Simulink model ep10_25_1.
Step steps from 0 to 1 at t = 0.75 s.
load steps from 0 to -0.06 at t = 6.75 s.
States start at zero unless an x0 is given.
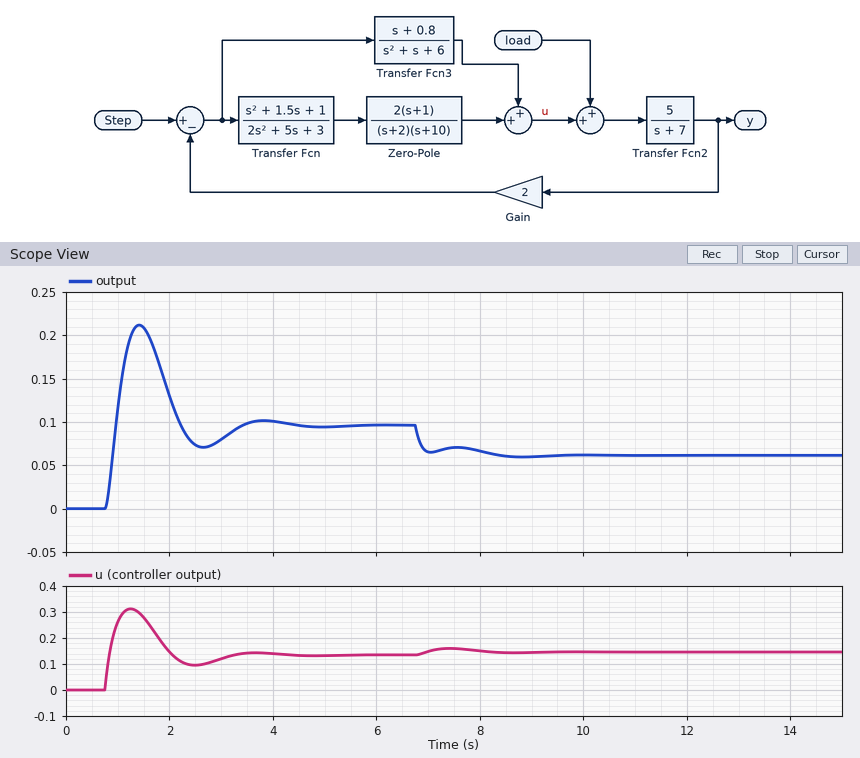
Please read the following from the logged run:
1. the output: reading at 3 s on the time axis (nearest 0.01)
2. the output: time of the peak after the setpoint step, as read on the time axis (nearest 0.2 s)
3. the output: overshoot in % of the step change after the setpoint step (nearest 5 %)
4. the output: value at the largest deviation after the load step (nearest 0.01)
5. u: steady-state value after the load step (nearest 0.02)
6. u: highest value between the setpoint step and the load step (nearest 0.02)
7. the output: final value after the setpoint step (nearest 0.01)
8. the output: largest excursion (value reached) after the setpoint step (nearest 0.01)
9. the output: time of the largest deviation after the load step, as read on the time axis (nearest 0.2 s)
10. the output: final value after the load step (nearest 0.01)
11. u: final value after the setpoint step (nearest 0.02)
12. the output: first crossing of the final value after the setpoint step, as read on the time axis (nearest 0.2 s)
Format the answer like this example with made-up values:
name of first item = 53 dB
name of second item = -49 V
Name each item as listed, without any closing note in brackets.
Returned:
the output: reading at 3 s on the time axis = 0.08
the output: time of the peak after the setpoint step, as read on the time axis = 1.4 s
the output: overshoot in % of the step change after the setpoint step = 120 %
the output: value at the largest deviation after the load step = 0.06
u: steady-state value after the load step = 0.14
u: highest value between the setpoint step and the load step = 0.32
the output: final value after the setpoint step = 0.10
the output: largest excursion (value reached) after the setpoint step = 0.21
the output: time of the largest deviation after the load step, as read on the time axis = 8.8 s
the output: final value after the load step = 0.06
u: final value after the setpoint step = 0.14
the output: first crossing of the final value after the setpoint step, as read on the time axis = 1.0 s
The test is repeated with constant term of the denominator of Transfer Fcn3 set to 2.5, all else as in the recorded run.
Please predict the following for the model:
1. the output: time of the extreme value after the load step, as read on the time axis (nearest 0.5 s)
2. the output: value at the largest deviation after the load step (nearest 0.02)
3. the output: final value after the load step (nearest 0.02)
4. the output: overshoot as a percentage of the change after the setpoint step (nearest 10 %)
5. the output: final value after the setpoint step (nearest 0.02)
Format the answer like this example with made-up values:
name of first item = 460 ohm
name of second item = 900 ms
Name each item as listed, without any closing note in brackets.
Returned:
the output: time of the extreme value after the load step, as read on the time axis = 7.0 s
the output: value at the largest deviation after the load step = 0.14
the output: final value after the load step = 0.14
the output: overshoot as a percentage of the change after the setpoint step = 60 %
the output: final value after the setpoint step = 0.16
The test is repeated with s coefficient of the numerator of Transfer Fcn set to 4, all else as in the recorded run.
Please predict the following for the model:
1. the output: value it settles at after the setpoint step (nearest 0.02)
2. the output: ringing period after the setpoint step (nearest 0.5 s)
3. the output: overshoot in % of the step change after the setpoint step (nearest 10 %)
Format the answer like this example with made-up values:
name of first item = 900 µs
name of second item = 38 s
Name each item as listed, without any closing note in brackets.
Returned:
the output: value it settles at after the setpoint step = 0.10
the output: ringing period after the setpoint step = 2.5 s
the output: overshoot in % of the step change after the setpoint step = 140 %
